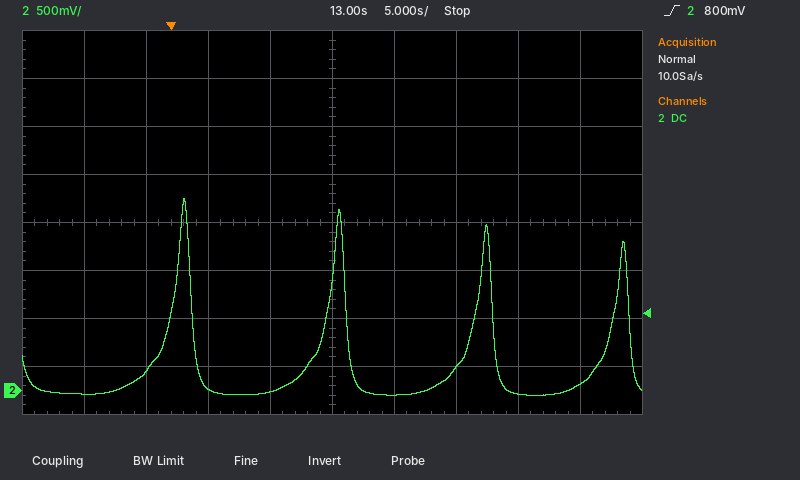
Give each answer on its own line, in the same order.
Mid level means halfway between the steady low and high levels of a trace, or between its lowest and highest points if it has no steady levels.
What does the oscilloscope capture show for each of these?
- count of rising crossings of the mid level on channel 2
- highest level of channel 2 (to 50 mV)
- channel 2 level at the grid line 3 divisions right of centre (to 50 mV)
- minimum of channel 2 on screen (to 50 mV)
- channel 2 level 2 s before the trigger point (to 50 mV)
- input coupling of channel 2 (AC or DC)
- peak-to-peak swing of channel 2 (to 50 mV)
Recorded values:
4
2.00 V
-50 mV
-50 mV
200 mV
DC
2.05 V
